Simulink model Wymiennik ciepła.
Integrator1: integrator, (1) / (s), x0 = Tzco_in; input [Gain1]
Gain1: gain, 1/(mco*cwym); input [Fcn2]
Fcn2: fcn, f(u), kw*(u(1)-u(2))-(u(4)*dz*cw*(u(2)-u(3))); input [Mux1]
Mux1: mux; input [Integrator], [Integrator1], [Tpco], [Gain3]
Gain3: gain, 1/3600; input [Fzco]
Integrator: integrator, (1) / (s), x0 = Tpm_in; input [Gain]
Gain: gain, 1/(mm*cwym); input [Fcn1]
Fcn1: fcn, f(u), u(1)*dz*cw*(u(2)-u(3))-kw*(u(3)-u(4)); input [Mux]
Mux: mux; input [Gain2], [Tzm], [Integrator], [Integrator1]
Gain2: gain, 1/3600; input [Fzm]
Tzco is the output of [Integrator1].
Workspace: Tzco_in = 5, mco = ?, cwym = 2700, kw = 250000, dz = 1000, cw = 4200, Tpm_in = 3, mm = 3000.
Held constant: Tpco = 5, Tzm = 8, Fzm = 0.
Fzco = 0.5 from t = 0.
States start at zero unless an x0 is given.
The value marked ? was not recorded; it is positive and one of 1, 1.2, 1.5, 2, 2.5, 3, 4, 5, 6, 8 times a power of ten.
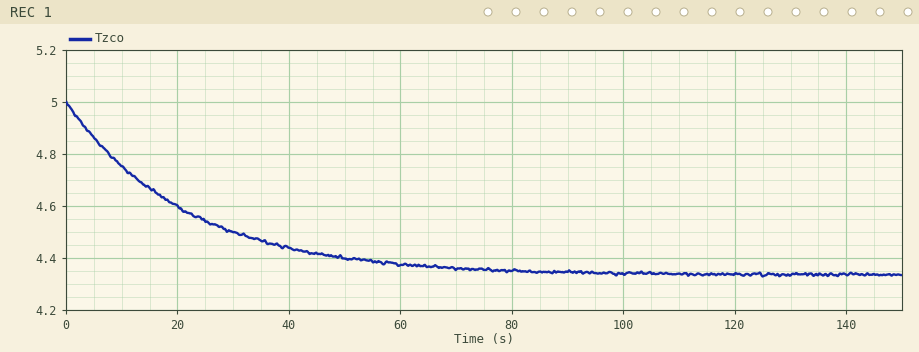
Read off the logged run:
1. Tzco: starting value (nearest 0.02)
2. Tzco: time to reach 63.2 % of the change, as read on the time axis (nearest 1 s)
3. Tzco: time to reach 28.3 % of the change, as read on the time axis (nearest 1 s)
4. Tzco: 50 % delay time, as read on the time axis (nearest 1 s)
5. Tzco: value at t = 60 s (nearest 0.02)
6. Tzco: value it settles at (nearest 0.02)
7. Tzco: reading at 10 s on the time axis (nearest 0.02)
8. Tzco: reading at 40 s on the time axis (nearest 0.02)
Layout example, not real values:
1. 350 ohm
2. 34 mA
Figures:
1. 5.00
2. 21 s
3. 7 s
4. 15 s
5. 4.38
6. 4.34
7. 4.76
8. 4.44
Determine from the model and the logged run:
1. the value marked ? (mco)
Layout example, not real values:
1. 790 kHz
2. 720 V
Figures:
1. 6000
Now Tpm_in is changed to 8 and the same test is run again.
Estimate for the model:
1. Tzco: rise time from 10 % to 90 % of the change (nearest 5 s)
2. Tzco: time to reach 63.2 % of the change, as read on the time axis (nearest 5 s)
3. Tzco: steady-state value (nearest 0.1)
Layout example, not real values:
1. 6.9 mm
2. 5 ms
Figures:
1. 45 s
2. 20 s
3. 6.0
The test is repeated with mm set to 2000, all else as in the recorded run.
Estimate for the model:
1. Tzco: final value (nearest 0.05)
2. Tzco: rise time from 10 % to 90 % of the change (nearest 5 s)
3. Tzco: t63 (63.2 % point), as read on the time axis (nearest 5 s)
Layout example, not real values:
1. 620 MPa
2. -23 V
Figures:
1. 4.50
2. 35 s
3. 15 s
